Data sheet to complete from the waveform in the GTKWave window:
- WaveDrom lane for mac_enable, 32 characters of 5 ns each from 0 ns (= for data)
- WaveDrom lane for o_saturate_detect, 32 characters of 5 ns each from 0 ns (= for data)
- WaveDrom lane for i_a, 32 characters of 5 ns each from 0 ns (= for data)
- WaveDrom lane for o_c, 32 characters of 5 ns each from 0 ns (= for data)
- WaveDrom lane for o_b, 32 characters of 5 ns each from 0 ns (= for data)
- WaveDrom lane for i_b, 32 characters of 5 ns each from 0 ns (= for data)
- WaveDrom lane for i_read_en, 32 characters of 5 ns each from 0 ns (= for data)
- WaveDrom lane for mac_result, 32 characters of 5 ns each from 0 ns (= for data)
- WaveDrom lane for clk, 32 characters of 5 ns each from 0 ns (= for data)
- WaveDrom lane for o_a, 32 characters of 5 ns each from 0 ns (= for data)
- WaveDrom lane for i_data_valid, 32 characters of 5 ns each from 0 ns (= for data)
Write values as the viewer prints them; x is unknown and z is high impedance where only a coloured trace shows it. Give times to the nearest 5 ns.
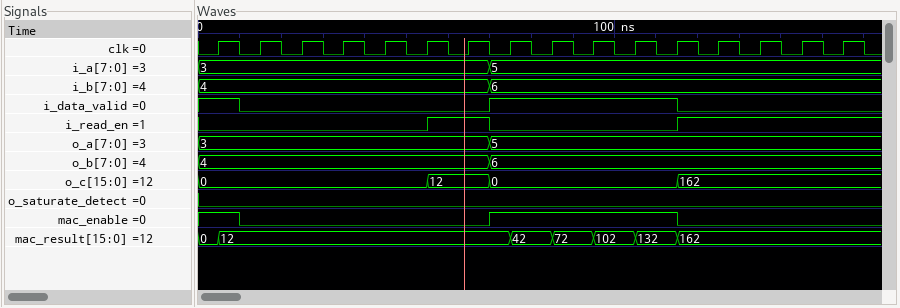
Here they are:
{name: 'mac_enable', wave: '1.0...........1........0........'}
{name: 'o_saturate_detect', wave: '0...............................'}
{name: 'i_a', wave: '=.............=.................', data: '3 5'}
{name: 'o_c', wave: '=..........=..=........=........', data: '0 12 0 162'}
{name: 'o_b', wave: '=.............=.................', data: '4 6'}
{name: 'i_b', wave: '=.............=.................', data: '4 6'}
{name: 'i_read_en', wave: '0..........1..0........1........'}
{name: 'mac_result', wave: '==.............=.=.=.=.=........', data: '0 12 42 72 102 132 162'}
{name: 'clk', wave: '01010101010101010101010101010101'}
{name: 'o_a', wave: '=.............=.................', data: '3 5'}
{name: 'i_data_valid', wave: '1.0...........1........0........'}
